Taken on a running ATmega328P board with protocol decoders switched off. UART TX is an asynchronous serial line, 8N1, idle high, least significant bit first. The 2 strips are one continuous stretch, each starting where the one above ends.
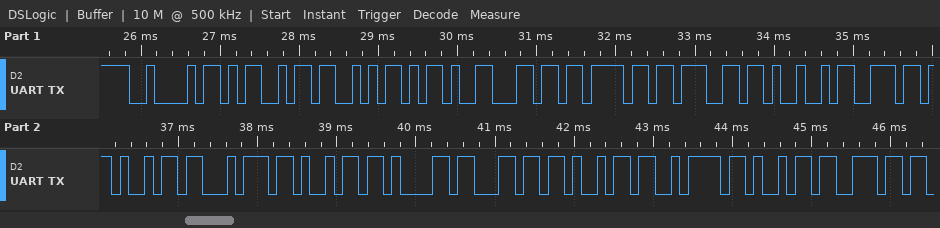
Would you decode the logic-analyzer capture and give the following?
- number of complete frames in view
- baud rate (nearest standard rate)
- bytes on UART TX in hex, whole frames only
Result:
18
9600 baud
0x42 0x4D 0x53 0x2D 0x6C 0x6F 0x67 0x49 0x6E 0x69 0x74 0x69 0x61 0x6C 0x69 0x7A 0x69 0x6E
